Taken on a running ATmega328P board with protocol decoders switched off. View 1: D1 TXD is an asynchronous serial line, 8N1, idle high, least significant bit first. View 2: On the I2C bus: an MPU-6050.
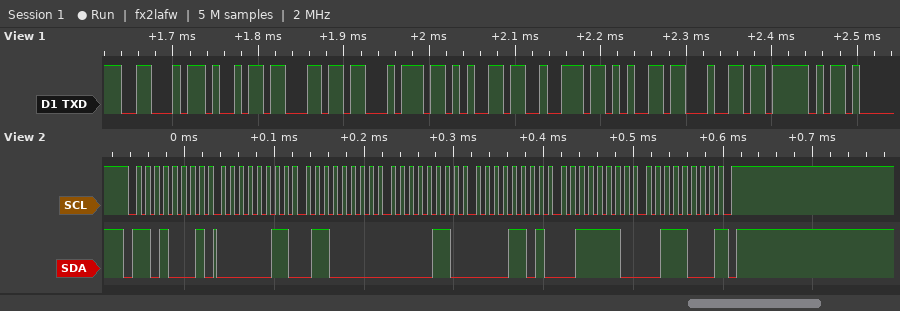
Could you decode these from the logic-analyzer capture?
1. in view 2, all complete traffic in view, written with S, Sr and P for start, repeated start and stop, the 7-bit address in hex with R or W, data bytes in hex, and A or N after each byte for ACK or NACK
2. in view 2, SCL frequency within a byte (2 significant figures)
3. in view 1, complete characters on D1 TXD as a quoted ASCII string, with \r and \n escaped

S 68R A 03 A 60 A 06 A 0D A 3E A 38 N P
100 kHz
"Filtered_"
